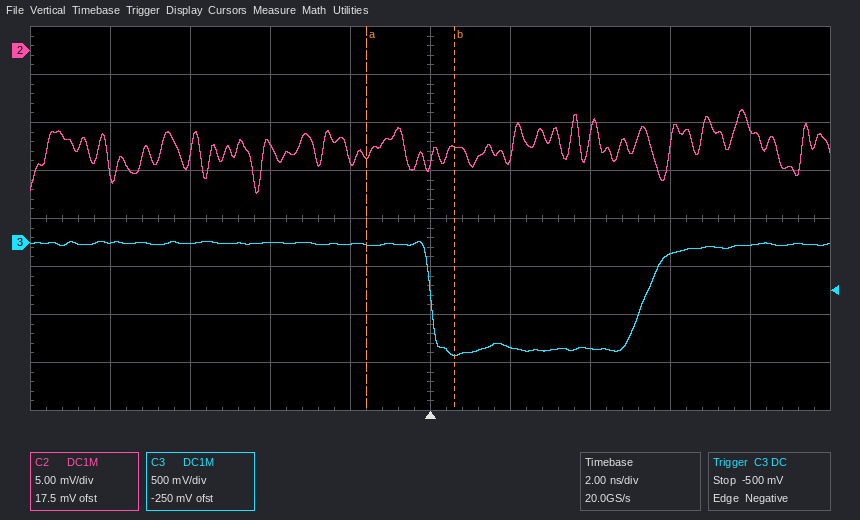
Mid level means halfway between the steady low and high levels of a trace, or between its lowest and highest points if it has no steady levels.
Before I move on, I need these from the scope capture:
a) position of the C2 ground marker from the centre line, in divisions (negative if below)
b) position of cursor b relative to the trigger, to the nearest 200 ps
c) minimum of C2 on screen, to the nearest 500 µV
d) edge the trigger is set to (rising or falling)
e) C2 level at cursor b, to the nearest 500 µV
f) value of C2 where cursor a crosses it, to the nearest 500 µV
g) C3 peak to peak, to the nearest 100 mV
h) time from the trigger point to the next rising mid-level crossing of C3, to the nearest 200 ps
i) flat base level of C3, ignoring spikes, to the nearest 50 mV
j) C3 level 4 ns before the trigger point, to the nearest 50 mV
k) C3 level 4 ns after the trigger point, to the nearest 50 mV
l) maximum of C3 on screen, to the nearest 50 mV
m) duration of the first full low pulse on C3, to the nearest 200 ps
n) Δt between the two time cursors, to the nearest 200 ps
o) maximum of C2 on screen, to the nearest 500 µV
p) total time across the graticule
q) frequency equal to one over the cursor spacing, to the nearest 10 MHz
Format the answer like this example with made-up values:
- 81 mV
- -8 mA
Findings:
- +3.5 div
- +600 ps
- -15.0 mV
- falling
- -10.0 mV
- -11.0 mV
- 1.20 V
- 5.4 ns
- -1.10 V
- 0 mV
- -1.10 V
- 0 mV
- 5.4 ns
- 2.2 ns
- -6.0 mV
- 20 ns
- 450 MHz
